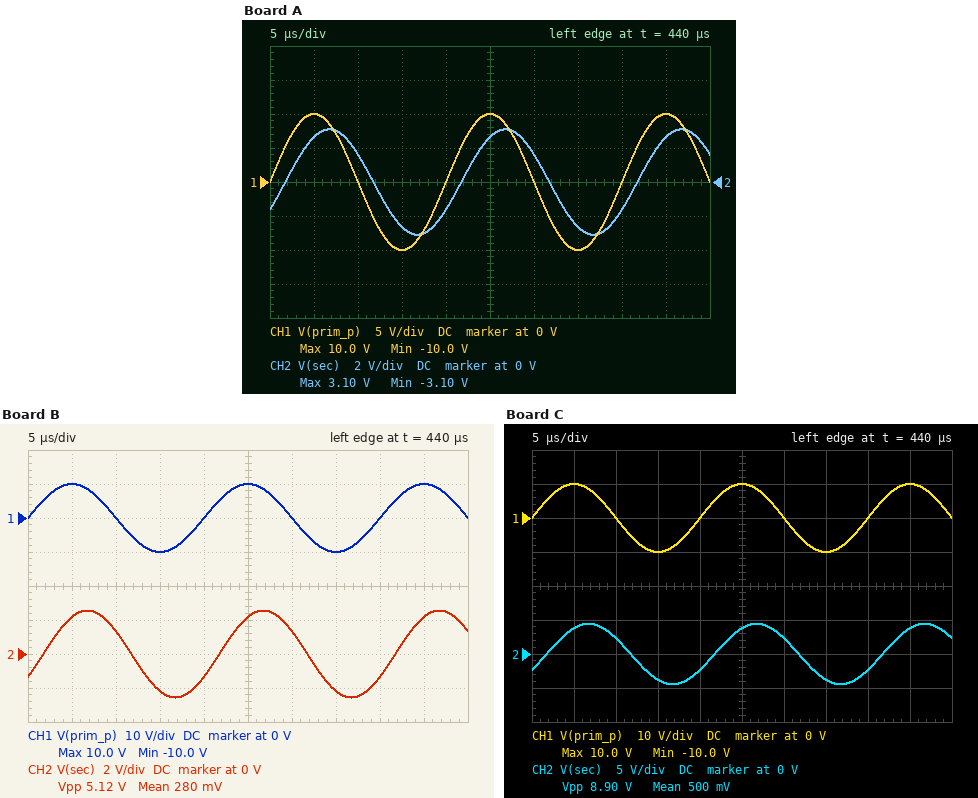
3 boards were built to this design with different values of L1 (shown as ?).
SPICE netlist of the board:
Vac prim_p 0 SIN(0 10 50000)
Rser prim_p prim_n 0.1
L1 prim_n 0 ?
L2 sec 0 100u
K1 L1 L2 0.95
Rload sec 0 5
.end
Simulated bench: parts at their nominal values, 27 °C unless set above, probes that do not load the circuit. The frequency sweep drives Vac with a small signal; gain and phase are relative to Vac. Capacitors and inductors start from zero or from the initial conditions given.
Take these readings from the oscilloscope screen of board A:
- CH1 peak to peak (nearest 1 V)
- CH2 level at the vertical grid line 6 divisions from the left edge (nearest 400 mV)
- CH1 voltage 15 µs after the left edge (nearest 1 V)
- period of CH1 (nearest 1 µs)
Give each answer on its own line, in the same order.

20 V
1.6 V
-10 V
20 µs
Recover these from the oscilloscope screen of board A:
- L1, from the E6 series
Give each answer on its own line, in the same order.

680 µH
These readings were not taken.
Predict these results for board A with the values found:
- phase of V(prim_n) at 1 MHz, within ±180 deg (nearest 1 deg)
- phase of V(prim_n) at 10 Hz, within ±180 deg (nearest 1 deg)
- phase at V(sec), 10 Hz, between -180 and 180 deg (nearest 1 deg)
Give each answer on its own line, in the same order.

0 deg
67 deg
67 deg
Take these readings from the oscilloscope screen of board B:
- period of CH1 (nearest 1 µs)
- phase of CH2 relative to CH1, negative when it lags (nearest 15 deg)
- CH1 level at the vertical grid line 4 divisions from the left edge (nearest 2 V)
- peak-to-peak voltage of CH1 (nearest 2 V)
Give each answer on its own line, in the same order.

20 µs
-30 deg
0 V
20 V
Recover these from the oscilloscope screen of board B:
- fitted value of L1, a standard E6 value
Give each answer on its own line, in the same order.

1 mH
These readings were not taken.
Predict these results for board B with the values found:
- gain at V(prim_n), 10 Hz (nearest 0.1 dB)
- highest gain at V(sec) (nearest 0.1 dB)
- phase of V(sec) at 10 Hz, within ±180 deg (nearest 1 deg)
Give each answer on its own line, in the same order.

-5.5 dB
-10.5 dB
58 deg
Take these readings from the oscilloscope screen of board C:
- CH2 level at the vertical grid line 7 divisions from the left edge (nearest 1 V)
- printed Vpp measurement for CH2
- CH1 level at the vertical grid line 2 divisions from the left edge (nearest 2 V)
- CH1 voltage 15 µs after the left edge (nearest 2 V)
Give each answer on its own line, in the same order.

-4 V
8.90 V
0 V
-10 V
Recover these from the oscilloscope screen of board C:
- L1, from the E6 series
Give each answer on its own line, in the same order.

330 µH
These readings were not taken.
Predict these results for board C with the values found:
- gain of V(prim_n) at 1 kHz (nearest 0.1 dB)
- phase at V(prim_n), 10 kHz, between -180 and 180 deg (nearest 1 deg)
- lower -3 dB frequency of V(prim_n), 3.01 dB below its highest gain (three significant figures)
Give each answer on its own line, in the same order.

-0.1 dB
0 deg
48.5 Hz
